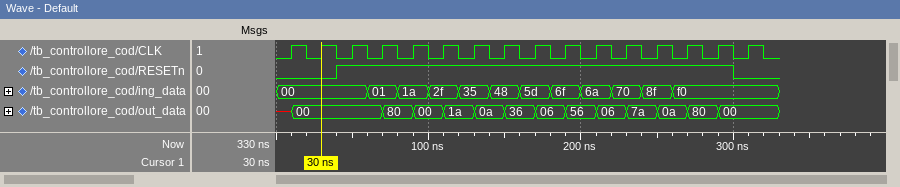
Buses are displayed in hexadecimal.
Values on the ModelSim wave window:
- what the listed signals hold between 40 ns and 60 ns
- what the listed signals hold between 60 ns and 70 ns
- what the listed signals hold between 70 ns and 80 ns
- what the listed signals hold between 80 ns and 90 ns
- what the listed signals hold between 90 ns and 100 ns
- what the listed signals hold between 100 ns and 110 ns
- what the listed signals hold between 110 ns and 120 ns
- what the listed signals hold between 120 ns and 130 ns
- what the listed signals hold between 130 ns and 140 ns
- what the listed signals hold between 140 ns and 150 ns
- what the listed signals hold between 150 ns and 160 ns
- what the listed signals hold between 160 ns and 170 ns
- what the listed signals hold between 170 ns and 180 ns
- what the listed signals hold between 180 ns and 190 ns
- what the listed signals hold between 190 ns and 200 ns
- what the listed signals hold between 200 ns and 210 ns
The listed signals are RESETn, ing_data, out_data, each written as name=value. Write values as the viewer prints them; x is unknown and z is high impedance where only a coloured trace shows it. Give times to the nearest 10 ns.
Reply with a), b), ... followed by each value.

a) RESETn=1, ing_data=00, out_data=00
b) RESETn=1, ing_data=01, out_data=00
c) RESETn=1, ing_data=01, out_data=80
d) RESETn=1, ing_data=1a, out_data=80
e) RESETn=1, ing_data=1a, out_data=00
f) RESETn=1, ing_data=2f, out_data=00
g) RESETn=1, ing_data=2f, out_data=1a
h) RESETn=1, ing_data=35, out_data=1a
i) RESETn=1, ing_data=35, out_data=0a
j) RESETn=1, ing_data=48, out_data=0a
k) RESETn=1, ing_data=48, out_data=36
l) RESETn=1, ing_data=5d, out_data=36
m) RESETn=1, ing_data=5d, out_data=06
n) RESETn=1, ing_data=6f, out_data=06
o) RESETn=1, ing_data=6f, out_data=56
p) RESETn=1, ing_data=6a, out_data=56
